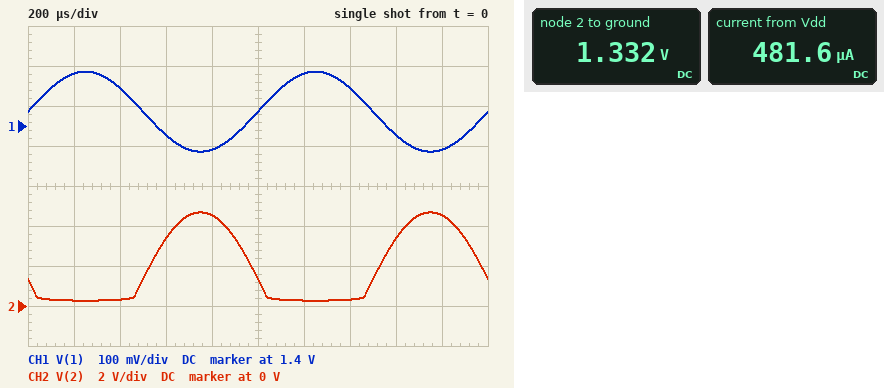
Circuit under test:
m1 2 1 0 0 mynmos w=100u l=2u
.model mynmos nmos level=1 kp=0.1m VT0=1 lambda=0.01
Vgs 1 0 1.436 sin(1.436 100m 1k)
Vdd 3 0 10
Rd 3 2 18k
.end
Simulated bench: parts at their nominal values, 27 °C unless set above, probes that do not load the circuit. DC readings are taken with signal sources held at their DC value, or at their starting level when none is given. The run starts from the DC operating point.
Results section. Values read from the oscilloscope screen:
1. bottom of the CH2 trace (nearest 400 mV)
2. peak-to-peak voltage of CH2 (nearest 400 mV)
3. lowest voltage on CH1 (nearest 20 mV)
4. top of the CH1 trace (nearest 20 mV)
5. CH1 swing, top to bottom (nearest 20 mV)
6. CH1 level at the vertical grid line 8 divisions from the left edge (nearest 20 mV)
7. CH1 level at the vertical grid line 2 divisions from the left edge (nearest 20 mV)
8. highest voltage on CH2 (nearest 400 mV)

400 mV
4.4 V
1.34 V
1.54 V
200 mV
1.38 V
1.50 V
4.8 V
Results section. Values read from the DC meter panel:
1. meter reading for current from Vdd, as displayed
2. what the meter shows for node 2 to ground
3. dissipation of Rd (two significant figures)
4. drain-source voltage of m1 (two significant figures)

481.6 µA
1.332 V
4.2 mW
1.3 V
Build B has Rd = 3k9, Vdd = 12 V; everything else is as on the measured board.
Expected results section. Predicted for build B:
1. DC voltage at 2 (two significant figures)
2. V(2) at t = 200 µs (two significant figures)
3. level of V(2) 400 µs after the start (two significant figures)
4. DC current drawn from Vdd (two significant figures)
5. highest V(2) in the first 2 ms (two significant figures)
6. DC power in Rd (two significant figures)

10 V
9.0 V
9.4 V
520 µA
11 V
1.1 mW
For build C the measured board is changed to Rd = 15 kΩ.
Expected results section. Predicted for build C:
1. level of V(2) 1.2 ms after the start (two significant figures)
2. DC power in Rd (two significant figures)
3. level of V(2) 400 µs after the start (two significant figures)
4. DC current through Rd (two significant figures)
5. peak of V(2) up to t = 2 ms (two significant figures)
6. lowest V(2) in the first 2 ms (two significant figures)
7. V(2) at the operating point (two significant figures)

370 mV
3.6 mW
750 mV
490 µA
5.5 V
360 mV
2.7 V
